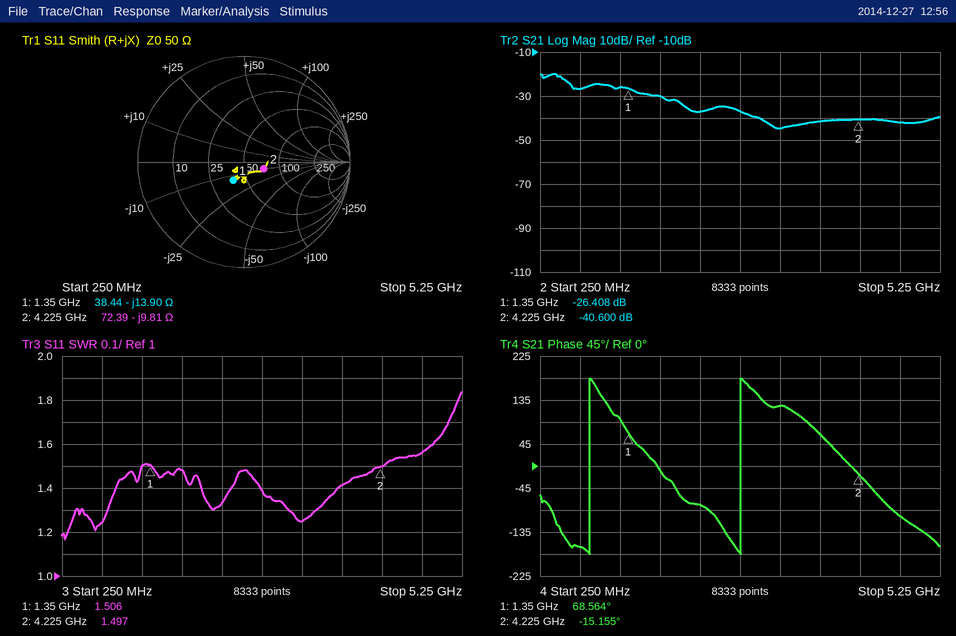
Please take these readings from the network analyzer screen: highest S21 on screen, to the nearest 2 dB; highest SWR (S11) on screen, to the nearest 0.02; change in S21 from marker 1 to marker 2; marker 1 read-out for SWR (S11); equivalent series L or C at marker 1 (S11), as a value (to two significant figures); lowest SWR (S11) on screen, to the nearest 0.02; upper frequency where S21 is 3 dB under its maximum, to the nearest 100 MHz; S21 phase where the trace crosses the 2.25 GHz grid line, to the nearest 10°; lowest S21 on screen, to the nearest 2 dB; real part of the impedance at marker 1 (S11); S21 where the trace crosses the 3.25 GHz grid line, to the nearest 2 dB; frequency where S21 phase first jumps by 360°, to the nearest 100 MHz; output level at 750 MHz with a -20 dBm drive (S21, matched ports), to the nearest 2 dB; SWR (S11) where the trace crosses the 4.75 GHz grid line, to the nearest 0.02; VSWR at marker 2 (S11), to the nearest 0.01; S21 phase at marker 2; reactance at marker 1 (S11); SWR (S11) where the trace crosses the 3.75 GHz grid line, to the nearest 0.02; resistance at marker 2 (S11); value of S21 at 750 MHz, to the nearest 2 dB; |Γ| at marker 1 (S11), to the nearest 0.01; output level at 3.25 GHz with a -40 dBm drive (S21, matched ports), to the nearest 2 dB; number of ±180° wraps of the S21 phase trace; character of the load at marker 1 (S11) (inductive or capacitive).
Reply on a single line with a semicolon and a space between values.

-20 dB; 1.84; -14.192 dB; 1.506; 8.5 pF; 1.16; 600 MHz; -80°; -44 dB; 38.44 Ω; -44 dB; 900 MHz; -46 dBm; 1.56; 1.50; -15.155°; -13.90 Ω; 1.42; 72.39 Ω; -26 dB; 0.20; -84 dBm; 2; capacitive
